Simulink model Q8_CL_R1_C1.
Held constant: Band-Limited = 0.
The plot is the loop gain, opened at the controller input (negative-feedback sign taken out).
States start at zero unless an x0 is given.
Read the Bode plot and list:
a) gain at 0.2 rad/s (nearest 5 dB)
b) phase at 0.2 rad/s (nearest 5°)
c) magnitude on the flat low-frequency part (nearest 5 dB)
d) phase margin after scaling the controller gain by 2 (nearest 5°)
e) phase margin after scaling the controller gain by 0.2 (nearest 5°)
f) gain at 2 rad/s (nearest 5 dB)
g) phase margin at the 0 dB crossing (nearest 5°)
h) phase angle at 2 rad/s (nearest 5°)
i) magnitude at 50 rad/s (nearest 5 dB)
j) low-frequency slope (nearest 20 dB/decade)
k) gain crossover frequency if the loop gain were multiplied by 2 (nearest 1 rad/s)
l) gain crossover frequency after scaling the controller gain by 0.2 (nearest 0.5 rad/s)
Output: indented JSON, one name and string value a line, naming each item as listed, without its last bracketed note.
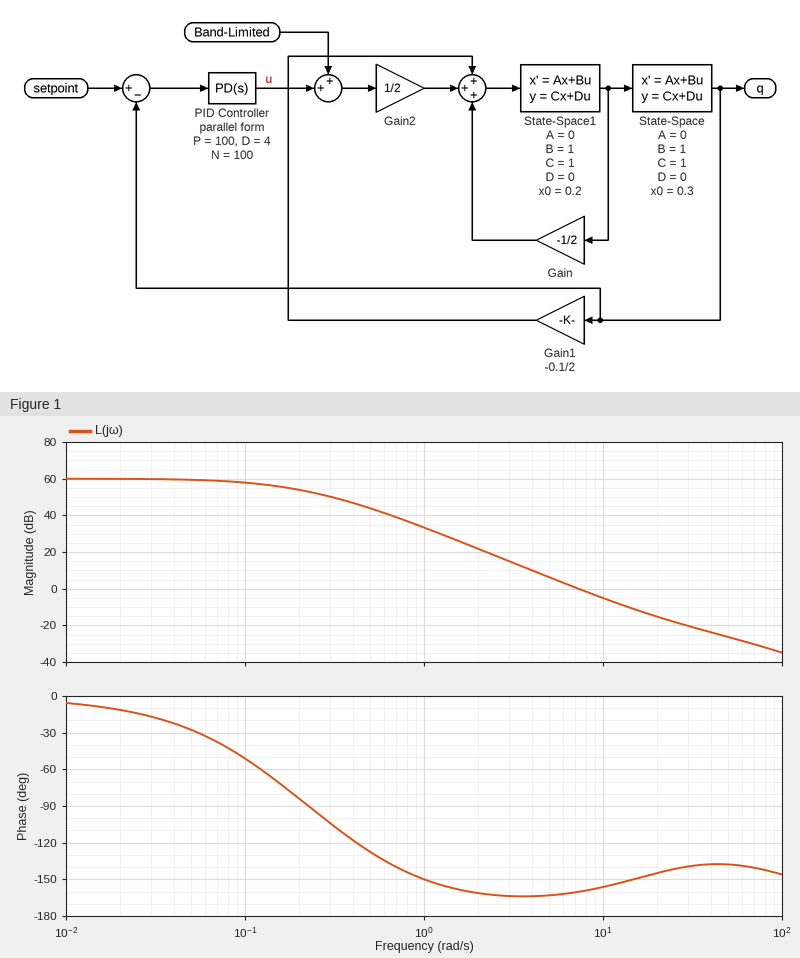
{
  "gain at 0.2 rad/s": "55 dB",
  "phase at 0.2 rad/s": "-85°",
  "magnitude on the flat low-frequency part": "60 dB",
  "phase margin after scaling the controller gain by 2": "25°",
  "phase margin after scaling the controller gain by 0.2": "15°",
  "gain at 2 rad/s": "20 dB",
  "phase margin at the 0 dB crossing": "20°",
  "phase angle at 2 rad/s": "-160°",
  "magnitude at 50 rad/s": "-25 dB",
  "low-frequency slope": "0 dB/decade",
  "gain crossover frequency if the loop gain were multiplied by 2": "11 rad/s",
  "gain crossover frequency after scaling the controller gain by 0.2": "3.0 rad/s"
}
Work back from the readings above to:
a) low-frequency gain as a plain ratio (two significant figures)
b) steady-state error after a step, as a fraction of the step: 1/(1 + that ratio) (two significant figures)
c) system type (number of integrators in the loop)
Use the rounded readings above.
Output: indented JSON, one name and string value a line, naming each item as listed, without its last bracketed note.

{
  "low-frequency gain as a plain ratio": "1000",
  "steady-state error after a step, as a fraction of the step: 1/(1 + that ratio)": "0.00100",
  "system type": "0"
}
